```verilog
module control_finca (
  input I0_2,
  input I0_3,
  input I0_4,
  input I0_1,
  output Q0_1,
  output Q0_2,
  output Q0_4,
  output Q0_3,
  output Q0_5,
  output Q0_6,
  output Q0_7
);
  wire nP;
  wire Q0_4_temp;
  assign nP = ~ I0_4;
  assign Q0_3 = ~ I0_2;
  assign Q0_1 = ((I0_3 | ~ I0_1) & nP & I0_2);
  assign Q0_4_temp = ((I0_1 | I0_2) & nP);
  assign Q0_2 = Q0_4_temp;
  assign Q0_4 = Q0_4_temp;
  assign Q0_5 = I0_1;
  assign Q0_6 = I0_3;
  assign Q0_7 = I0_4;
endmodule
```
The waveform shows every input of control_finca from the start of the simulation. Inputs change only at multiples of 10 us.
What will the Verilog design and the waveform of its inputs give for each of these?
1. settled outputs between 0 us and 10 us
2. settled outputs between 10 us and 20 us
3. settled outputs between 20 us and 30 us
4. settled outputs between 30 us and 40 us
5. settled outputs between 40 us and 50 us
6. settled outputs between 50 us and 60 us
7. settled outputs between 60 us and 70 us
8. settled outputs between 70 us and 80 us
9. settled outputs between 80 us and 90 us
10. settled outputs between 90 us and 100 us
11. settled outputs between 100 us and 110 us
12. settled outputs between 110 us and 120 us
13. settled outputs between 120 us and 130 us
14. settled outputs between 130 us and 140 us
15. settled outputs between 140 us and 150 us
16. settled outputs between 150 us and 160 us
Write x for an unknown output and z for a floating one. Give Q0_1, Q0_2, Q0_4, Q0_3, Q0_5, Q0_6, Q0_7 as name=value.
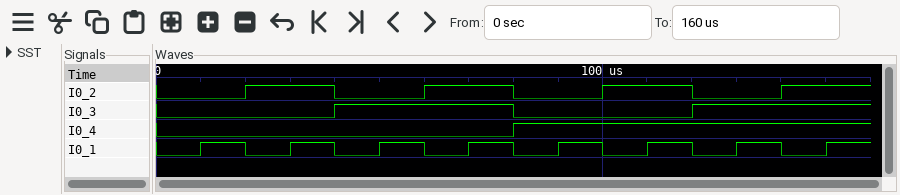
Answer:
Q0_1=0, Q0_2=0, Q0_4=0, Q0_3=1, Q0_5=0, Q0_6=0, Q0_7=0
Q0_1=0, Q0_2=1, Q0_4=1, Q0_3=1, Q0_5=1, Q0_6=0, Q0_7=0
Q0_1=1, Q0_2=1, Q0_4=1, Q0_3=0, Q0_5=0, Q0_6=0, Q0_7=0
Q0_1=0, Q0_2=1, Q0_4=1, Q0_3=0, Q0_5=1, Q0_6=0, Q0_7=0
Q0_1=0, Q0_2=0, Q0_4=0, Q0_3=1, Q0_5=0, Q0_6=1, Q0_7=0
Q0_1=0, Q0_2=1, Q0_4=1, Q0_3=1, Q0_5=1, Q0_6=1, Q0_7=0
Q0_1=1, Q0_2=1, Q0_4=1, Q0_3=0, Q0_5=0, Q0_6=1, Q0_7=0
Q0_1=1, Q0_2=1, Q0_4=1, Q0_3=0, Q0_5=1, Q0_6=1, Q0_7=0
Q0_1=0, Q0_2=0, Q0_4=0, Q0_3=1, Q0_5=0, Q0_6=0, Q0_7=1
Q0_1=0, Q0_2=0, Q0_4=0, Q0_3=1, Q0_5=1, Q0_6=0, Q0_7=1
Q0_1=0, Q0_2=0, Q0_4=0, Q0_3=0, Q0_5=0, Q0_6=0, Q0_7=1
Q0_1=0, Q0_2=0, Q0_4=0, Q0_3=0, Q0_5=1, Q0_6=0, Q0_7=1
Q0_1=0, Q0_2=0, Q0_4=0, Q0_3=1, Q0_5=0, Q0_6=1, Q0_7=1
Q0_1=0, Q0_2=0, Q0_4=0, Q0_3=1, Q0_5=1, Q0_6=1, Q0_7=1
Q0_1=0, Q0_2=0, Q0_4=0, Q0_3=0, Q0_5=0, Q0_6=1, Q0_7=1
Q0_1=0, Q0_2=0, Q0_4=0, Q0_3=0, Q0_5=1, Q0_6=1, Q0_7=1
